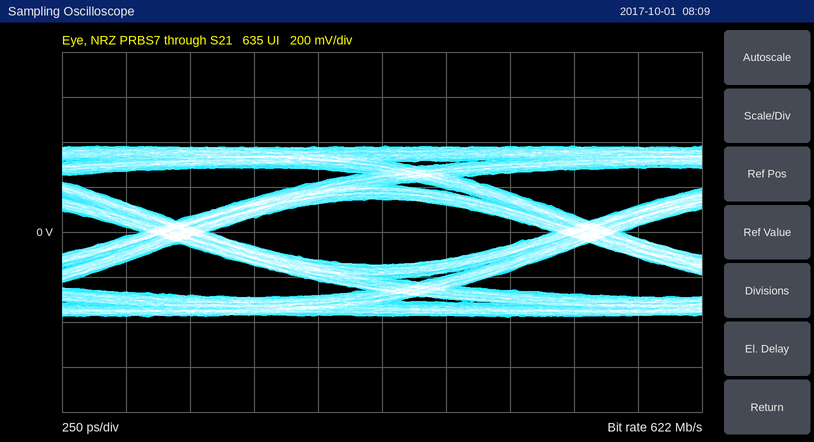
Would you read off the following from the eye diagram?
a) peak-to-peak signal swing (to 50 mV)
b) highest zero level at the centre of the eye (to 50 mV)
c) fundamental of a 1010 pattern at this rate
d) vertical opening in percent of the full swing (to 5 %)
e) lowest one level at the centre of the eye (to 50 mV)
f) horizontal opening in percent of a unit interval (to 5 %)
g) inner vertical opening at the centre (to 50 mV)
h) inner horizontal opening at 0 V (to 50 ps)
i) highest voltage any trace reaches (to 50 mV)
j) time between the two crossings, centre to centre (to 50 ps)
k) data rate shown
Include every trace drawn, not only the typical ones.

750 mV
-150 mV
311 MHz
40 %
150 mV
85 %
300 mV
1.35 ns
400 mV
1.60 ns
622 Mb/s
